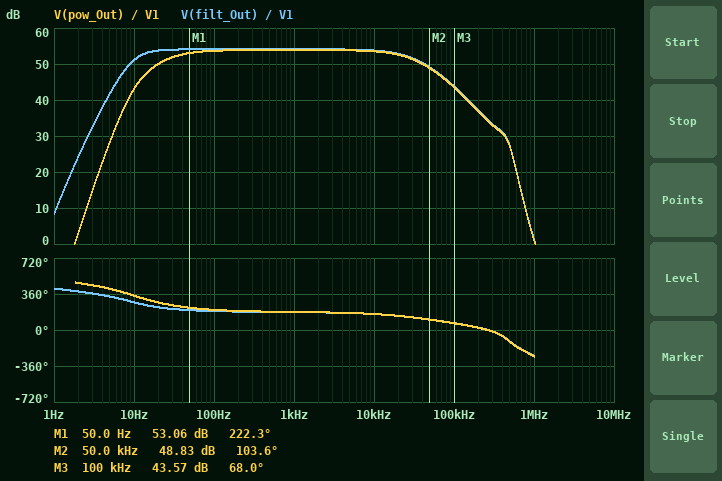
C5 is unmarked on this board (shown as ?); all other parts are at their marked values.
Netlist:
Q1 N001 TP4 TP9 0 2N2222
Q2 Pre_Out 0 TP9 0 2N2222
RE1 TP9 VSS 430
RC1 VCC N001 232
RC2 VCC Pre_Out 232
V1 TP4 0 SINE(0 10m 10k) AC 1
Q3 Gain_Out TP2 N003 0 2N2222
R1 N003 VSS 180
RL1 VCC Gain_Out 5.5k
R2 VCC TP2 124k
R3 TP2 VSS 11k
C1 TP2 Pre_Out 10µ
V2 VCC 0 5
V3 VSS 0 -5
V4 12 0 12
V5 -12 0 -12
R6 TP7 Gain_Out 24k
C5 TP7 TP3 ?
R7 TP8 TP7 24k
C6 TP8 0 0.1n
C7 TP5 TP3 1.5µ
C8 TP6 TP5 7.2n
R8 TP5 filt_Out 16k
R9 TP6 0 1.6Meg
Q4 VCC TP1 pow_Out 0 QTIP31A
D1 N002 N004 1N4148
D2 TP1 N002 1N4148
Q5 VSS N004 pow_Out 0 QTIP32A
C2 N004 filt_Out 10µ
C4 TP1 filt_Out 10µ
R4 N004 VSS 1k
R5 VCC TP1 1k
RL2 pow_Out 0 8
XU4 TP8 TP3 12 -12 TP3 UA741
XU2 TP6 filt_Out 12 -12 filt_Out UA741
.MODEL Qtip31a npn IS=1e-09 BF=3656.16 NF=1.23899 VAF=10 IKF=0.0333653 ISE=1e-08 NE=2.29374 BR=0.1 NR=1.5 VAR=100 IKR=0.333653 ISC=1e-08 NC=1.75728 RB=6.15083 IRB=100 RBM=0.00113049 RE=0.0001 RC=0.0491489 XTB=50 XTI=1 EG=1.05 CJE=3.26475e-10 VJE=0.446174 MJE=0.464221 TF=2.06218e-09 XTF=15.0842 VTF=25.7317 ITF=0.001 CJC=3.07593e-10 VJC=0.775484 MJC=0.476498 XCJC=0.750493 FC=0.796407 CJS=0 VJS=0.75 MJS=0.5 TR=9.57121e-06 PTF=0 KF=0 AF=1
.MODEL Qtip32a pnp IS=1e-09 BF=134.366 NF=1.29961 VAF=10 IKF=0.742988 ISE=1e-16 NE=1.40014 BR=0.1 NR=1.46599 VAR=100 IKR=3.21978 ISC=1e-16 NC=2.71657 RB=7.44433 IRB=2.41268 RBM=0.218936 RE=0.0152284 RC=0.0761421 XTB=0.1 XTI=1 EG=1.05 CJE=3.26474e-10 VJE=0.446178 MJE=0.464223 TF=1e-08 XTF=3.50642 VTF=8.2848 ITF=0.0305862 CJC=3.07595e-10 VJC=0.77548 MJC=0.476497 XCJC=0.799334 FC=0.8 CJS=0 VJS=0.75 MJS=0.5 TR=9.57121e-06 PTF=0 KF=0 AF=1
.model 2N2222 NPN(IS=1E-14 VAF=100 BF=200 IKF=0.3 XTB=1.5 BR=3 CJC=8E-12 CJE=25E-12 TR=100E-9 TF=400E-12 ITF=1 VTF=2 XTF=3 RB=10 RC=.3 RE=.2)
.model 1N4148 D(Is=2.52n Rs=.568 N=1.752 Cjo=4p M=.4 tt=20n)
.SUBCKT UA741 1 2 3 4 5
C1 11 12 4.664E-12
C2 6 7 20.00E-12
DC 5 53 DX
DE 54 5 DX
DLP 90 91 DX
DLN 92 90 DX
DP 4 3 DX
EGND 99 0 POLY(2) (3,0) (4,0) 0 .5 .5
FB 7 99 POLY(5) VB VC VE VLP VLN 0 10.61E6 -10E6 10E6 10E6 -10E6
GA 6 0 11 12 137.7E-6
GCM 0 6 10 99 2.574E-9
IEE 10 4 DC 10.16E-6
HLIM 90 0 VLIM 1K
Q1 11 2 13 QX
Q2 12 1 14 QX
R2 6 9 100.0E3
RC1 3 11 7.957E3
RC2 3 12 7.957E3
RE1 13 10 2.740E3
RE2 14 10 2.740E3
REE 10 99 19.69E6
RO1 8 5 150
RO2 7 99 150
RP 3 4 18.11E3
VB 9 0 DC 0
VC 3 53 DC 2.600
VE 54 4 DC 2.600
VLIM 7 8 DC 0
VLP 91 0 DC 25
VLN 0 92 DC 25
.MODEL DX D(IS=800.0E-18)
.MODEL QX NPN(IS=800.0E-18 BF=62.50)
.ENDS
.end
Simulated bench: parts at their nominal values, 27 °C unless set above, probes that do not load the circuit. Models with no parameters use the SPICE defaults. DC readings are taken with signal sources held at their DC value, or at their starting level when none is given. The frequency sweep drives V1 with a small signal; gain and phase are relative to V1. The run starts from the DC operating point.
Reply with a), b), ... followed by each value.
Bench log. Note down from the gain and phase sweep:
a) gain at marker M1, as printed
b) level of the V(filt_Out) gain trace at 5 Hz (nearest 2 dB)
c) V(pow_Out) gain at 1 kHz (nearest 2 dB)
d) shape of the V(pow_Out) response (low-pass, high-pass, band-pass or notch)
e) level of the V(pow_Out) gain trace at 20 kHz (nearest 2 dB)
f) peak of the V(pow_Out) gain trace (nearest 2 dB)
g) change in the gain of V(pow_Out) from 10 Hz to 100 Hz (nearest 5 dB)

a) 53.06 dB
b) 42 dB
c) 54 dB
d) band-pass
e) 52 dB
f) 54 dB
g) 10 dB
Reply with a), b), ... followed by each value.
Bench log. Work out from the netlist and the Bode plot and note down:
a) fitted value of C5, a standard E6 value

a) 47 pF
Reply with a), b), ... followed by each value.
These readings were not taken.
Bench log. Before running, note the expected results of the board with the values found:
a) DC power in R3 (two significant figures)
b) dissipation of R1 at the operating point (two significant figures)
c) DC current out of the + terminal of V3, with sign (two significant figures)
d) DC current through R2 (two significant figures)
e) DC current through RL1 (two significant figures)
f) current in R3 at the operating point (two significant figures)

a) 55 µW
b) 99 µW
c) -170 mA
d) 74 µA
e) 740 µA
f) 71 µA
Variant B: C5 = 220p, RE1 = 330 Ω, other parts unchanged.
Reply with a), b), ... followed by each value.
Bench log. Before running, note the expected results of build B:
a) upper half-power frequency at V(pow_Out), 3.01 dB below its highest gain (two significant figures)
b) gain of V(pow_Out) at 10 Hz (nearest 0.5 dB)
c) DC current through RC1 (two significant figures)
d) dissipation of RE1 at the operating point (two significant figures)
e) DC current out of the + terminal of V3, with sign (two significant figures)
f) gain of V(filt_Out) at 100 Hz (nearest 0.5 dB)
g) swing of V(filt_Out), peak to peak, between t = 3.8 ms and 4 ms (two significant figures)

a) 42 kHz
b) 45.0 dB
c) 6.5 mA
d) 56 mW
e) -180 mA
f) 56.0 dB
g) 9.8 V
